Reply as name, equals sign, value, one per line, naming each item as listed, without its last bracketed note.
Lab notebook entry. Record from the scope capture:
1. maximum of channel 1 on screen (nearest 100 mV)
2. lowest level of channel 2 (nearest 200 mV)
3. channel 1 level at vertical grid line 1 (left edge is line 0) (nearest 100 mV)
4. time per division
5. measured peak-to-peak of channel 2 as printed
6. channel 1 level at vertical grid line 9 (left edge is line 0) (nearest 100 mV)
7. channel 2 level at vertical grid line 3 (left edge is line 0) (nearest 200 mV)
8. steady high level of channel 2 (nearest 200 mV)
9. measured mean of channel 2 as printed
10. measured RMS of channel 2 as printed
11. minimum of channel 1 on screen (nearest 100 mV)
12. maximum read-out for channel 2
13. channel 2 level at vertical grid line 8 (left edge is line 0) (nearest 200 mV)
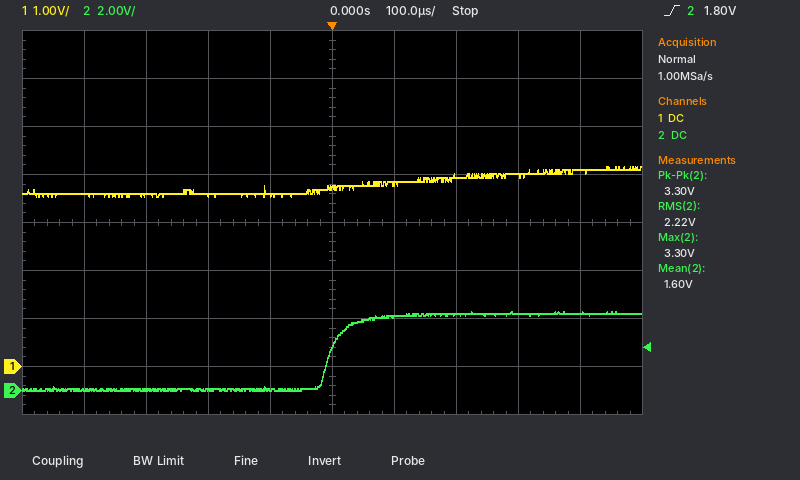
maximum of channel 1 on screen = 4.2 V
lowest level of channel 2 = 0.0 V
channel 1 level at vertical grid line 1 (left edge is line 0) = 3.6 V
time per division = 100 µs
measured peak-to-peak of channel 2 as printed = 3.30 V
channel 1 level at vertical grid line 9 (left edge is line 0) = 4.1 V
channel 2 level at vertical grid line 3 (left edge is line 0) = 0.0 V
steady high level of channel 2 = 3.2 V
measured mean of channel 2 as printed = 1.60 V
measured RMS of channel 2 as printed = 2.22 V
minimum of channel 1 on screen = 3.5 V
maximum read-out for channel 2 = 3.30 V
channel 2 level at vertical grid line 8 (left edge is line 0) = 3.2 V
